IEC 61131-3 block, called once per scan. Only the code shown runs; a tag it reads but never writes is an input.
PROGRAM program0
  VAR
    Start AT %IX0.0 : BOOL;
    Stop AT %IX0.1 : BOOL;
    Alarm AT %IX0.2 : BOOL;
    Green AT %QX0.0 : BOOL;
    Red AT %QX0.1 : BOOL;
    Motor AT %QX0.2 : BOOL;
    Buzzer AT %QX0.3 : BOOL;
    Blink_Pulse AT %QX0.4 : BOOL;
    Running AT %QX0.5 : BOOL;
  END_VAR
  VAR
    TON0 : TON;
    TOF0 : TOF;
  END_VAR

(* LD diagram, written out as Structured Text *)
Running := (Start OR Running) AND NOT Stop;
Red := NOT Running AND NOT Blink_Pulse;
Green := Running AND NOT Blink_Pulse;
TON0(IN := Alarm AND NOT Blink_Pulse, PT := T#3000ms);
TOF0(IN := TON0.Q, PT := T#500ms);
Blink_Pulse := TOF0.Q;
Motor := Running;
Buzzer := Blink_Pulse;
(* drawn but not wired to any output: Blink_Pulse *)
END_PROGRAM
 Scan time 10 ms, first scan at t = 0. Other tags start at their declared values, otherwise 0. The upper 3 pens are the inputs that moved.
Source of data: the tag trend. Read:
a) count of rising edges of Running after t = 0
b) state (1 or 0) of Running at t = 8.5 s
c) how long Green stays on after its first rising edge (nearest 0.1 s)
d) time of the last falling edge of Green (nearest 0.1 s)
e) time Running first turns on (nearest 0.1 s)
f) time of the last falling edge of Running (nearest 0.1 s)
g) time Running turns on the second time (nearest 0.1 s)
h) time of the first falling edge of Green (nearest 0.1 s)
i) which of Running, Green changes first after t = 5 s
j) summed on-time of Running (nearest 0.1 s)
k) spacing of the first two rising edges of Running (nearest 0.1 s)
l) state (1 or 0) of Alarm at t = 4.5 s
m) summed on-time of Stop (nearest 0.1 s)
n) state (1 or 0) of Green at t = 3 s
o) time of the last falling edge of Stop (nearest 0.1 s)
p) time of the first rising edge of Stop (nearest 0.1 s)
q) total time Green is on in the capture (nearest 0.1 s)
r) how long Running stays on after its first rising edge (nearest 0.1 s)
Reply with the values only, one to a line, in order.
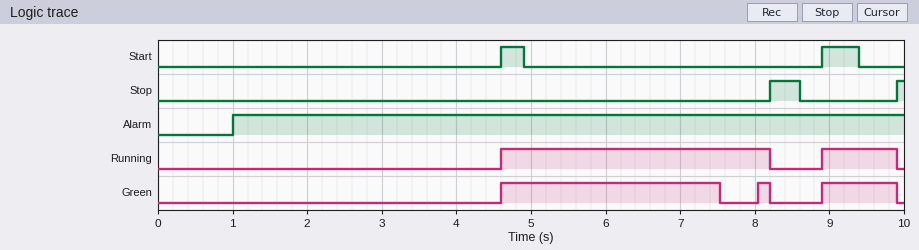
2
0
2.9 s
9.9 s
4.6 s
9.9 s
8.9 s
7.5 s
Green
4.6 s
4.3 s
1
0.5 s
0
8.6 s
8.2 s
4.1 s
3.6 s
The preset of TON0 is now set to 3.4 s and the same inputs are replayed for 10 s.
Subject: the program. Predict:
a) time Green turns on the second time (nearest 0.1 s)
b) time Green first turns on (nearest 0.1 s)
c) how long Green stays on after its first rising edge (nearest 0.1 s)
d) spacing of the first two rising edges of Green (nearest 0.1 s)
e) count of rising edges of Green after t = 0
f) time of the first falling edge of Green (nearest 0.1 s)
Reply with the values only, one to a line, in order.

8.9 s
4.9 s
3.3 s
4.0 s
2
8.2 s
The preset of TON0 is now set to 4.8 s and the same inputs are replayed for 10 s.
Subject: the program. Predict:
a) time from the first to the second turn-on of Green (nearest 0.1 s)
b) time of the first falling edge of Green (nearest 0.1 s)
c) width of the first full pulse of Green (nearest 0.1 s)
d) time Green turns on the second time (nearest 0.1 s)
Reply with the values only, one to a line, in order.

1.7 s
5.8 s
1.2 s
6.3 s
